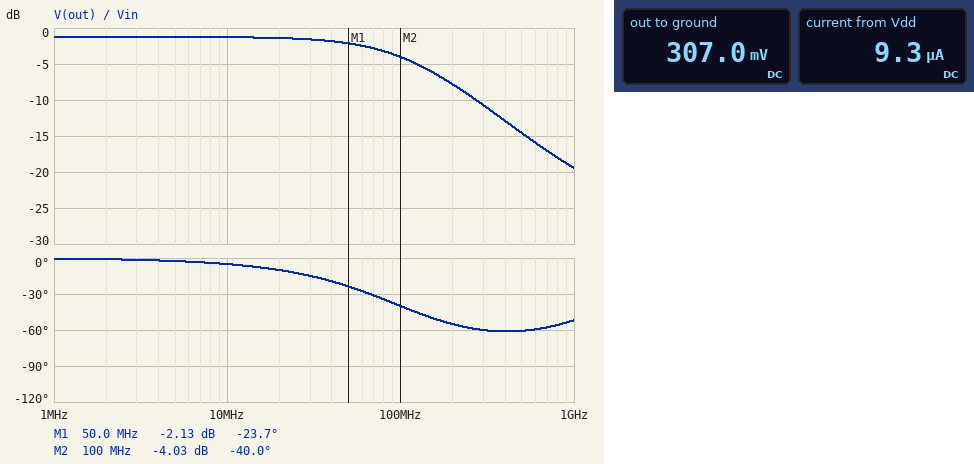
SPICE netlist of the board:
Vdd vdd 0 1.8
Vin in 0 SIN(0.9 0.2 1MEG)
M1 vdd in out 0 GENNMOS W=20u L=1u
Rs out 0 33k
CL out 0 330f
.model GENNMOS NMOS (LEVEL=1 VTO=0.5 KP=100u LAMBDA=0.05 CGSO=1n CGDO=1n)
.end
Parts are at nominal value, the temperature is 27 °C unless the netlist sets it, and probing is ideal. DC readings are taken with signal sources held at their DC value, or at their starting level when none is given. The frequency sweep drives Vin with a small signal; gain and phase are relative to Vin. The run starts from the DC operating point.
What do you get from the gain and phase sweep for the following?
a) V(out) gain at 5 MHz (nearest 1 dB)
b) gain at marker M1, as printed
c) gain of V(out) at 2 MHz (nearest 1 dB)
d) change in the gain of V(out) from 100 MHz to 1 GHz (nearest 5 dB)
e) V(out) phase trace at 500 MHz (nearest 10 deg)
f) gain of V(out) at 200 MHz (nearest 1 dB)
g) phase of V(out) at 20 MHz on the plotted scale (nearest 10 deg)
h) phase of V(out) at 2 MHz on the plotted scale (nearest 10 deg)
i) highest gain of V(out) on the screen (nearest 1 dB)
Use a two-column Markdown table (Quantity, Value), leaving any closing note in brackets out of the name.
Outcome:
| Quantity | Value |
|---|---|
| V(out) gain at 5 MHz | -1 dB |
| gain at marker M1, as printed | -2.13 dB |
| gain of V(out) at 2 MHz | -1 dB |
| change in the gain of V(out) from 100 MHz to 1 GHz | -15 dB |
| V(out) phase trace at 500 MHz | -60 deg |
| gain of V(out) at 200 MHz | -8 dB |
| phase of V(out) at 20 MHz on the plotted scale | -10 deg |
| phase of V(out) at 2 MHz on the plotted scale | 0 deg |
| highest gain of V(out) on the screen | -1 dB |
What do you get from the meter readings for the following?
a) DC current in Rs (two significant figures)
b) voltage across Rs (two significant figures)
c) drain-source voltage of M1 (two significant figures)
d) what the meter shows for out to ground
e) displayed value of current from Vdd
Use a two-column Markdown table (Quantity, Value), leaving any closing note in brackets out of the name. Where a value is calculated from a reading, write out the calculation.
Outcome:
| Quantity | Value |
|---|---|
| DC current in Rs | (307 mV) / 33 kΩ = 9.3 µA |
| voltage across Rs | 307 mV = 310 mV |
| drain-source voltage of M1 | 1.8 V - 307 mV = 1.5 V |
| what the meter shows for out to ground | 307.0 mV |
| displayed value of current from Vdd | 9.3 µA |
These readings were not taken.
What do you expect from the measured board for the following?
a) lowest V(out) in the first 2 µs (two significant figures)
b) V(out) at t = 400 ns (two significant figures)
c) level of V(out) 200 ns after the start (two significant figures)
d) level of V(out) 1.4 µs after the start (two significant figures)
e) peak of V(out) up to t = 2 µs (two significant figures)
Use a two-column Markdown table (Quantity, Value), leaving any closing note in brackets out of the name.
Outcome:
| Quantity | Value |
|---|---|
| lowest V(out) in the first 2 µs | 140 mV |
| V(out) at t = 400 ns | 410 mV |
| level of V(out) 200 ns after the start | 470 mV |
| level of V(out) 1.4 µs after the start | 410 mV |
| peak of V(out) up to t = 2 µs | 480 mV |
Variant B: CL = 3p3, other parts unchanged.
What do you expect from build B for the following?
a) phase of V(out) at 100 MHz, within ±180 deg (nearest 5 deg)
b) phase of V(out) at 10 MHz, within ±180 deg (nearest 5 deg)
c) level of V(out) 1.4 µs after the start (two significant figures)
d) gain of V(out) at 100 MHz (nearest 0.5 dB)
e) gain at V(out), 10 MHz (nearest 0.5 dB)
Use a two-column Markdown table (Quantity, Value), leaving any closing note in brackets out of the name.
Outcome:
| Quantity | Value |
|---|---|
| phase of V(out) at 100 MHz, within ±180 deg | -80 deg |
| phase of V(out) at 10 MHz, within ±180 deg | -40 deg |
| level of V(out) 1.4 µs after the start | 420 mV |
| gain of V(out) at 100 MHz | -20.5 dB |
| gain at V(out), 10 MHz | -4.0 dB |
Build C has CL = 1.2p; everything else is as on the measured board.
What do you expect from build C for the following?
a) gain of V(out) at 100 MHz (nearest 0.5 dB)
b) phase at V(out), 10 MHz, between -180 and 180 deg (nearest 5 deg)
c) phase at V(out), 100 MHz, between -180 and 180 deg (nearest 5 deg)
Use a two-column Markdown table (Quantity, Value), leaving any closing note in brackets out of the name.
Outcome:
| Quantity | Value |
|---|---|
| gain of V(out) at 100 MHz | -12.0 dB |
| phase at V(out), 10 MHz, between -180 and 180 deg | -20 deg |
| phase at V(out), 100 MHz, between -180 and 180 deg | -70 deg |
